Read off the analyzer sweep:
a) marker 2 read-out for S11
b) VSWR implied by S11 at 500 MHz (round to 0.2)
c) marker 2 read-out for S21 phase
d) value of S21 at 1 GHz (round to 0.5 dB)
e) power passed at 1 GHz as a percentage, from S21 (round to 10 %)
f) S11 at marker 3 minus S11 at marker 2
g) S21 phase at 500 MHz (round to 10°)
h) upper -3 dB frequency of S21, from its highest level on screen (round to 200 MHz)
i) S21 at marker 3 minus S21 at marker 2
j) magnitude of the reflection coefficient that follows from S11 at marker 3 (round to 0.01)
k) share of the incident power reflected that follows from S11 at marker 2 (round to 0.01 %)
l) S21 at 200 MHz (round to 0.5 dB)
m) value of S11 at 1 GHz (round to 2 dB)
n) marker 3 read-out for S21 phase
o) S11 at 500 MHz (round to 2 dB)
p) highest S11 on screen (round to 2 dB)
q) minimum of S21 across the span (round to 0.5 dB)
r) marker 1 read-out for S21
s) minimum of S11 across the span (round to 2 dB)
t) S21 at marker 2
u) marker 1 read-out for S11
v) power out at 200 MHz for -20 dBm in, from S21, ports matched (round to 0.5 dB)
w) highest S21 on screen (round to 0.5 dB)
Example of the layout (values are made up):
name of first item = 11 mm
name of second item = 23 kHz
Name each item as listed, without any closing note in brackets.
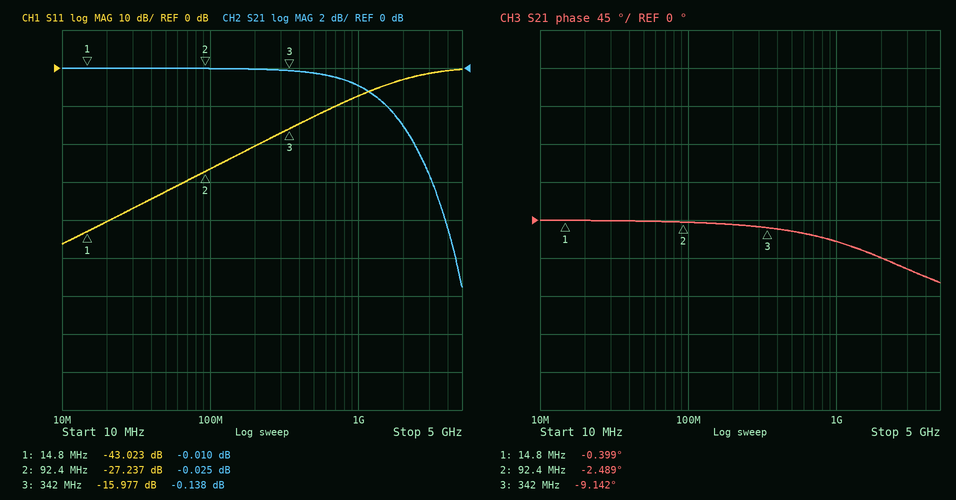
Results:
marker 2 read-out for S11 = -27.237 dB
VSWR implied by S11 at 500 MHz = 1.6
marker 2 read-out for S21 phase = -2.489°
value of S21 at 1 GHz = -1.0 dB
power passed at 1 GHz as a percentage, from S21 = 80 %
S11 at marker 3 minus S11 at marker 2 = 11.260 dB
S21 phase at 500 MHz = -10°
upper -3 dB frequency of S21, from its highest level on screen = 2.0 GHz
S21 at marker 3 minus S21 at marker 2 = -0.113 dB
magnitude of the reflection coefficient that follows from S11 at marker 3 = 0.16
share of the incident power reflected that follows from S11 at marker 2 = 0.19 %
S21 at 200 MHz = 0.0 dB
value of S11 at 1 GHz = -8 dB
marker 3 read-out for S21 phase = -9.142°
S11 at 500 MHz = -12 dB
highest S11 on screen = 0 dB
minimum of S21 across the span = -11.5 dB
marker 1 read-out for S21 = -0.010 dB
minimum of S11 across the span = -46 dB
S21 at marker 2 = -0.025 dB
marker 1 read-out for S11 = -43.023 dB
power out at 200 MHz for -20 dBm in, from S21, ports matched = -20.0 dBm
highest S21 on screen = 0.0 dB
